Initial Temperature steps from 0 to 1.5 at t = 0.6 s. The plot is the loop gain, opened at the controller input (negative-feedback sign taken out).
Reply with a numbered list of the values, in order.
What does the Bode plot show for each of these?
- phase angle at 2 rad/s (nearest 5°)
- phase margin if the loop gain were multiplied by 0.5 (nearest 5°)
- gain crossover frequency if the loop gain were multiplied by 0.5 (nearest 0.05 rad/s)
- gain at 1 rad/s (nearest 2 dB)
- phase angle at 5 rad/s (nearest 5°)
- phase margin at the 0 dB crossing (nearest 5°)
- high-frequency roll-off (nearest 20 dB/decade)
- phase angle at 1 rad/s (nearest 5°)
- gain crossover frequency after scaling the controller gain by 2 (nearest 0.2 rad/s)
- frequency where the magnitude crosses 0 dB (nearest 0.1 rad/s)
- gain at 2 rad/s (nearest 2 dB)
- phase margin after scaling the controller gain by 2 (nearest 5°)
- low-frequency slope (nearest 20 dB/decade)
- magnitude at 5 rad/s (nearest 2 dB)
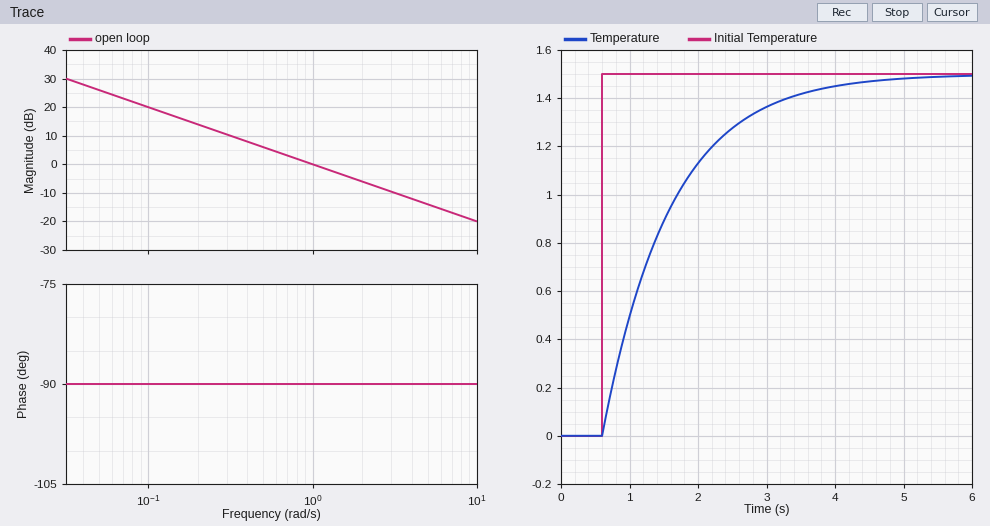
1. -90°
2. 90°
3. 0.50 rad/s
4. 0 dB
5. -90°
6. 90°
7. -20 dB/decade
8. -90°
9. 2.0 rad/s
10. 1.0 rad/s
11. -6 dB
12. 90°
13. -20 dB/decade
14. -14 dB
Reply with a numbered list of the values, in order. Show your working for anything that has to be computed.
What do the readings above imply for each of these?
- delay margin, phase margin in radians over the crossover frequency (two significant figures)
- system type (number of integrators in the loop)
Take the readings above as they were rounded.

1. 90 × π / 180 / 1 = 1.6 s
2. 1
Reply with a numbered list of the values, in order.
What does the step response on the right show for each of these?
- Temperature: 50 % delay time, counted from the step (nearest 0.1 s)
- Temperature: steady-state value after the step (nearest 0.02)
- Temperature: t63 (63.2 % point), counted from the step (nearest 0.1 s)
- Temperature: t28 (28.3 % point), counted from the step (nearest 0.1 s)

1. 0.7 s
2. 1.50
3. 1.0 s
4. 0.3 s
